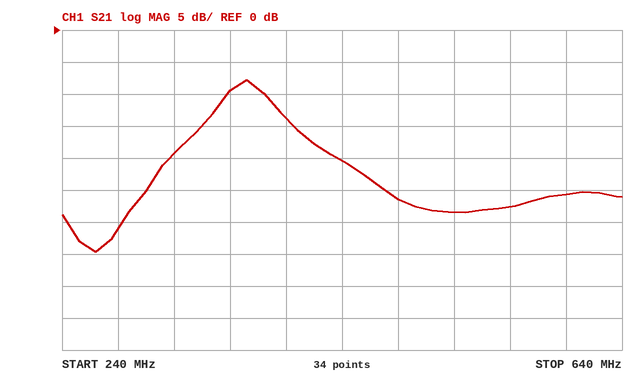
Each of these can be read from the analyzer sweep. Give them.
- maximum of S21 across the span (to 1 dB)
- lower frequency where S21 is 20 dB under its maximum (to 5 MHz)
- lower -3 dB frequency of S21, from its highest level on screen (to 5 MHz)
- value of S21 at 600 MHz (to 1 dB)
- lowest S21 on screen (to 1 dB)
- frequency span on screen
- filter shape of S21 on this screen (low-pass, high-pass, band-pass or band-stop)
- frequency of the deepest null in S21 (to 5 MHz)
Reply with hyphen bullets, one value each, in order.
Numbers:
- -8 dB
- 290 MHz
- 355 MHz
- -26 dB
- -35 dB
- 400 MHz
- band-pass
- 265 MHz
